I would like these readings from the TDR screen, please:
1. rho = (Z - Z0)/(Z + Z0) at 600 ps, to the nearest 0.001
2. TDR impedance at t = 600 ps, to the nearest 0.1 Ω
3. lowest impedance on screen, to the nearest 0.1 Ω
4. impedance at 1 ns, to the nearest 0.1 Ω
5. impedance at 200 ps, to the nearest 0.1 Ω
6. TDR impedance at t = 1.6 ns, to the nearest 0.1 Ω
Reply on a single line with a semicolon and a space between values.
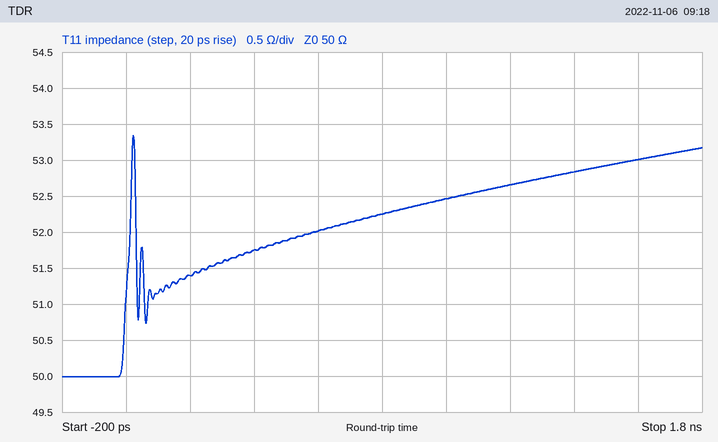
+0.020; 52.0 Ω; 50.0 Ω; 52.5 Ω; 51.4 Ω; 53.0 Ω
